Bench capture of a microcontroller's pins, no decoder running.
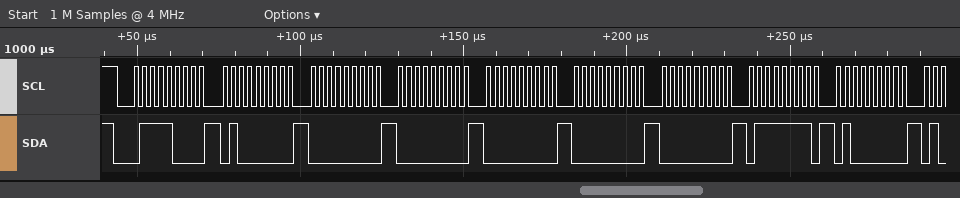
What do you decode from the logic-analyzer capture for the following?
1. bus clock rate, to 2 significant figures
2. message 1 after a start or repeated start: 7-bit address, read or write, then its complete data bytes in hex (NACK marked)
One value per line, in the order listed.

400 kHz
0x3C write: 40 00 00 00 00 00 7F 40
